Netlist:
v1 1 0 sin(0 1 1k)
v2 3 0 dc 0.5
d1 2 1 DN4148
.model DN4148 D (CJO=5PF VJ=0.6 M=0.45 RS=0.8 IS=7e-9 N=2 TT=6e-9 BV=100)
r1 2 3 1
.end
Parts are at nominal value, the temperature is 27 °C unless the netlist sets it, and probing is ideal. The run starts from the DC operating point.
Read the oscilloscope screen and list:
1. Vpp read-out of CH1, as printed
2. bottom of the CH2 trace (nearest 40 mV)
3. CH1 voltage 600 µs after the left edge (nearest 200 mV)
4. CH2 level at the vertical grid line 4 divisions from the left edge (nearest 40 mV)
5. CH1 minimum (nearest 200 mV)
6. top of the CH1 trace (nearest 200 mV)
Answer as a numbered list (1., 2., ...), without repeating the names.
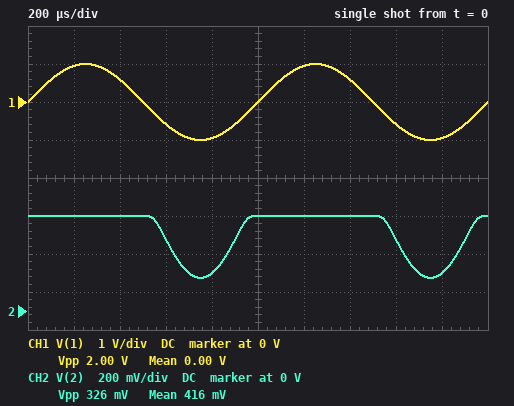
1. 2.00 V
2. 160 mV
3. -600 mV
4. 200 mV
5. -1.0 V
6. 1.0 V
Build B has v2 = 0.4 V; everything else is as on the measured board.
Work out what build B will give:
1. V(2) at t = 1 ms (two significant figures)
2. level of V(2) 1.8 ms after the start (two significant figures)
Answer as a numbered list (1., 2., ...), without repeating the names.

1. 400 mV
2. 150 mV
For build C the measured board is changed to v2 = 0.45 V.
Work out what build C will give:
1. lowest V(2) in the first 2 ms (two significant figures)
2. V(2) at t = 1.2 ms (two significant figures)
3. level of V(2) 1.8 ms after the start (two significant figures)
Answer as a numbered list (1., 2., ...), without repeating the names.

1. 150 mV
2. 450 mV
3. 170 mV
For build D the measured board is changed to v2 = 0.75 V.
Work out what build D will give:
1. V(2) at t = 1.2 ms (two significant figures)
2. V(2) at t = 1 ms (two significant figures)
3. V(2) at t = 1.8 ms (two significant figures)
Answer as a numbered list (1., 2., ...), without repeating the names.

1. 750 mV
2. 740 mV
3. 320 mV
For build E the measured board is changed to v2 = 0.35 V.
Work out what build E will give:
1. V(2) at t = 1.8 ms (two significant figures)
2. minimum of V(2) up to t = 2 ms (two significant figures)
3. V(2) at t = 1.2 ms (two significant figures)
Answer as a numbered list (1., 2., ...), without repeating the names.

1. 120 mV
2. 100 mV
3. 350 mV
